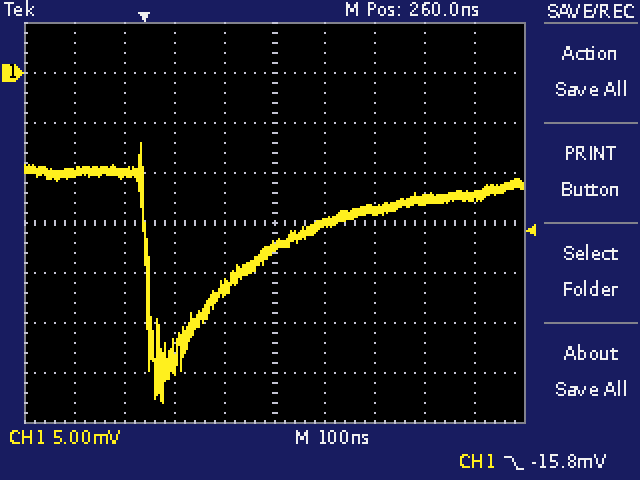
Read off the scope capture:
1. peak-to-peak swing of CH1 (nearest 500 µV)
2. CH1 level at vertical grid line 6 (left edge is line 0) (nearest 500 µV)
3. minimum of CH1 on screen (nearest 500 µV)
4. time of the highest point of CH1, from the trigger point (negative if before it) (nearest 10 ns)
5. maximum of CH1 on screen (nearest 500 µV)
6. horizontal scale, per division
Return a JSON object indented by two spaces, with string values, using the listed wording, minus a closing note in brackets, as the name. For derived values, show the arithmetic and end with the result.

{
  "peak-to-peak swing of CH1": "-7.0 mV − (-33.0 mV) = 26.0 mV",
  "CH1 level at vertical grid line 6 (left edge is line 0)": "-15.0 mV",
  "minimum of CH1 on screen": "-33.0 mV",
  "time of the highest point of CH1, from the trigger point (negative if before it)": "-10 ns",
  "maximum of CH1 on screen": "-7.0 mV",
  "horizontal scale, per division": "100 ns"
}
